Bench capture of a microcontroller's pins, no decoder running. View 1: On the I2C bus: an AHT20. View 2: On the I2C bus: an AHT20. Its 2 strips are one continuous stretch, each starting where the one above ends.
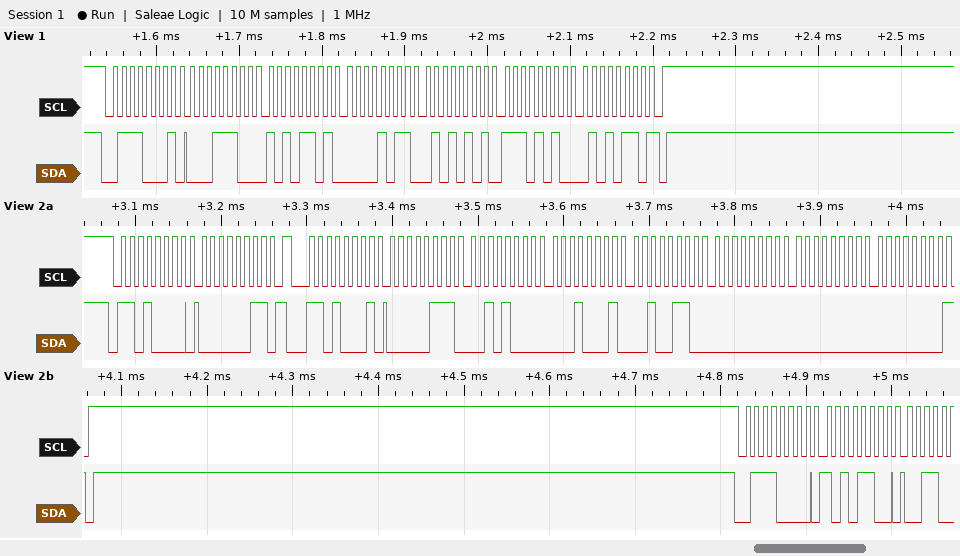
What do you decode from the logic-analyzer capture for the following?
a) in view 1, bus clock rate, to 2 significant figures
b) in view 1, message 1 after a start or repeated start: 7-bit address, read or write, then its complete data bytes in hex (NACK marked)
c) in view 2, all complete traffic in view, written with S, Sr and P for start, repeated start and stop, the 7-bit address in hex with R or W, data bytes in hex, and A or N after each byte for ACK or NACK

100 kHz
0x38 read: 1C AD 0B 55 EA 56 NACK
S 68W A 03 A Sr 68R A 07 A 28 A 11 A 26 A 00 A 00 A 00 N P S 38W A AC A
